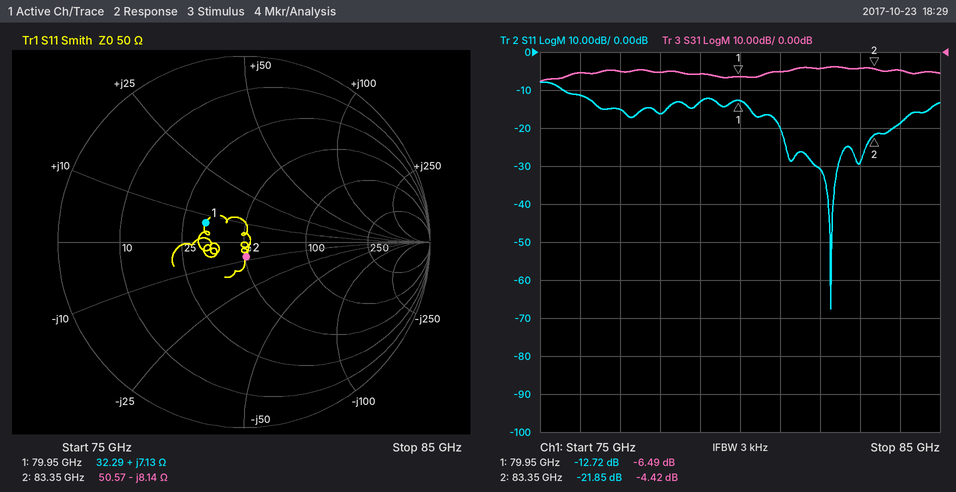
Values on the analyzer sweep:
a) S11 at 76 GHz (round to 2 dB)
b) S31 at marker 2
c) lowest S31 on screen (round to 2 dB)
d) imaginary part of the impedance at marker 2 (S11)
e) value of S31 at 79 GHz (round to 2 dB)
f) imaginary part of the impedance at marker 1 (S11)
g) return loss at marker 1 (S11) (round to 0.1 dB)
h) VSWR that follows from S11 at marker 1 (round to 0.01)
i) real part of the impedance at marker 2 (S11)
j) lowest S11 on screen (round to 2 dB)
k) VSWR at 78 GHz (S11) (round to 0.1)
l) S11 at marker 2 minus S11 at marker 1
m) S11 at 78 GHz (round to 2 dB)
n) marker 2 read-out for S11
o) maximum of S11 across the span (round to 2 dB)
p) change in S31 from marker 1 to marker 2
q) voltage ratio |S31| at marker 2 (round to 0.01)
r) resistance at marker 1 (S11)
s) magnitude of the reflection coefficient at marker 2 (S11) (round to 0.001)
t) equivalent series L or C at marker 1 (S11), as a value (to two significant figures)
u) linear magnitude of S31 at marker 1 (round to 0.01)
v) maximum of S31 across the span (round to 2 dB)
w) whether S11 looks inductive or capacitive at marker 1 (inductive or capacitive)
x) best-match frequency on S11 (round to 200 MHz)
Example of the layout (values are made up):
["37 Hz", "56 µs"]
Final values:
["-12 dB", "-4.42 dB", "-8 dB", "-8.14 Ω", "-6 dB", "+7.13 Ω", "12.7 dB", "1.60", "50.57 Ω", "-68 dB", "1.4", "-9.13 dB", "-16 dB", "-21.85 dB", "-8 dB", "2.07 dB", "0.60", "32.29 Ω", "0.081", "14 pH", "0.47", "-4 dB", "inductive", "82.2 GHz"]
